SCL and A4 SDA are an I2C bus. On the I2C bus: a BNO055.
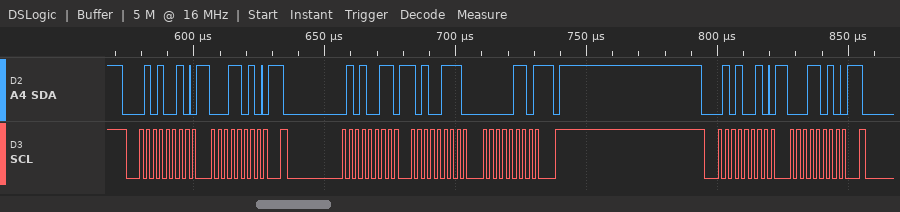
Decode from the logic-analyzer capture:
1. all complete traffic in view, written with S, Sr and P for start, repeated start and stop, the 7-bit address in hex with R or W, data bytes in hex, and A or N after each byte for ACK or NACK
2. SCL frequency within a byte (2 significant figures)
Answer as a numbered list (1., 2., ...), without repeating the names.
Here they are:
1. S 29W A 1A A Sr 29R A A7 A 06 N P S 29W A 1A A
2. 400 kHz
